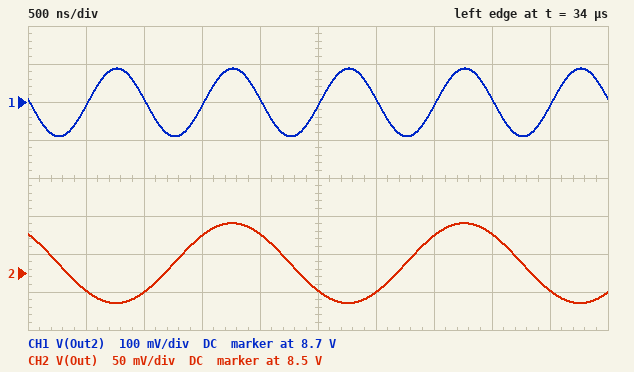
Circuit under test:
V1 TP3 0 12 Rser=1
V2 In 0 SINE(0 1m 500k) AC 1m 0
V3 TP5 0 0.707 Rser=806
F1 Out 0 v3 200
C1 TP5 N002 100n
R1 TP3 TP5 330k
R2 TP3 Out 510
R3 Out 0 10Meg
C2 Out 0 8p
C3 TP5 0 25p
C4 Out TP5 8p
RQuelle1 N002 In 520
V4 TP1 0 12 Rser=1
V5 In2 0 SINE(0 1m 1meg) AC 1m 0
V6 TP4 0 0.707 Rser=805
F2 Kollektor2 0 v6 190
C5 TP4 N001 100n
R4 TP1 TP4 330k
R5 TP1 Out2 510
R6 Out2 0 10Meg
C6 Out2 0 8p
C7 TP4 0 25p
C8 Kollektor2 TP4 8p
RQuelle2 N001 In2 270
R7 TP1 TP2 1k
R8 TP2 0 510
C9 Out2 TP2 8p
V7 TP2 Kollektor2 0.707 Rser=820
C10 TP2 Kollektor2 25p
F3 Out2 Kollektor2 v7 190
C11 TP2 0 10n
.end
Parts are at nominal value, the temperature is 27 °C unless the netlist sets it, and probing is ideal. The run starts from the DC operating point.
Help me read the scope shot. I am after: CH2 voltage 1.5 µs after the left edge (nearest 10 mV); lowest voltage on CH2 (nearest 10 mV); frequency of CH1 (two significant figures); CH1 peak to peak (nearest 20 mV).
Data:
8.55 V
8.46 V
1.0 MHz
180 mV
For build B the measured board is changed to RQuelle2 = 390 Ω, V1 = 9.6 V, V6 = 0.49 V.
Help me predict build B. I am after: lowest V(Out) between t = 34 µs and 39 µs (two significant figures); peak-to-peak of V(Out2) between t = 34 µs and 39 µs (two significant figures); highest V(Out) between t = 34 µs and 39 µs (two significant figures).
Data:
6.8 V
160 mV
6.9 V
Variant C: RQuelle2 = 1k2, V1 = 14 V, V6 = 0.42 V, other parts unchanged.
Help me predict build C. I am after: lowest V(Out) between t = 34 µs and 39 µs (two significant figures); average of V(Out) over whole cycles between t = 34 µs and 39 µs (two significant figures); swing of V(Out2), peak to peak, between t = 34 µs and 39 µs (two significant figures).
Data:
9.8 V
9.9 V
95 mV
